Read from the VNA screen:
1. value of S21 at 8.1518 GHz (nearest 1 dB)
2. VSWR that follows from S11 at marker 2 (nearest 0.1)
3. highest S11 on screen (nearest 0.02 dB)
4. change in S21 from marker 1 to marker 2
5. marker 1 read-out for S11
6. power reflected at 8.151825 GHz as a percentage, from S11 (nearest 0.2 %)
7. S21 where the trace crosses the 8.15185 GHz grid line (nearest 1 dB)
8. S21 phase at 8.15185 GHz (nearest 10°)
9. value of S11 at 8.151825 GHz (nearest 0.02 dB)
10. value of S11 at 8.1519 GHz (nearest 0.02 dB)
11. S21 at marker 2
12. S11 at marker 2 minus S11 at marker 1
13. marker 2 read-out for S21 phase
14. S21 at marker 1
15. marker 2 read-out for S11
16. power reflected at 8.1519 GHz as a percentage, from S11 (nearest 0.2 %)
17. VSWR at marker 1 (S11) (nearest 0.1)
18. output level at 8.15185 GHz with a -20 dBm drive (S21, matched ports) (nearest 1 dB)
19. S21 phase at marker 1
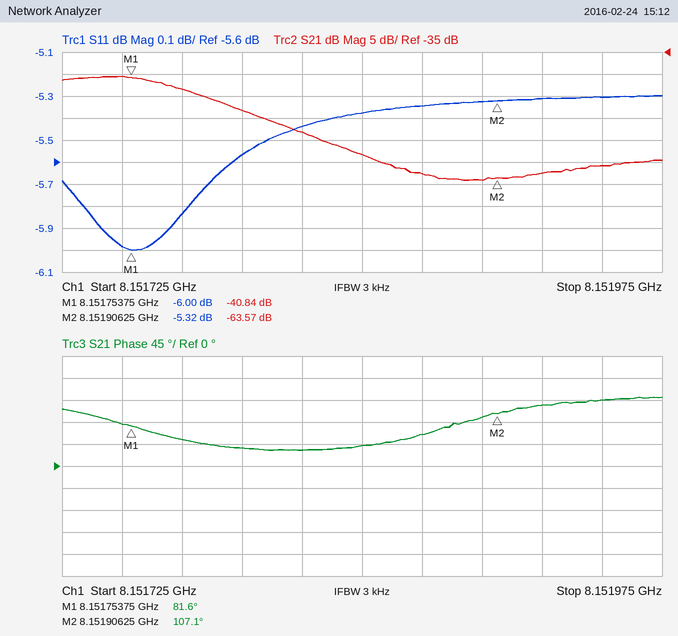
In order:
-48 dB
3.4
-5.30 dB
-22.73 dB
-6.00 dB
28.6 %
-58 dB
40°
-5.44 dB
-5.32 dB
-63.57 dB
0.68 dB
107.1°
-40.84 dB
-5.32 dB
29.4 %
3.0
-78 dBm
81.6°
